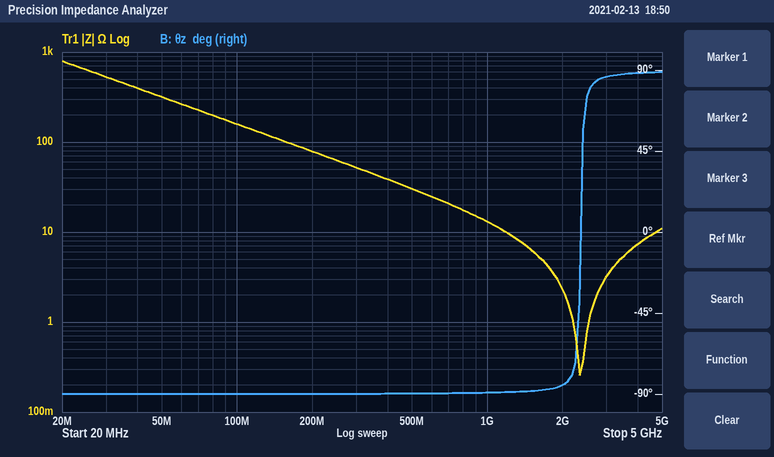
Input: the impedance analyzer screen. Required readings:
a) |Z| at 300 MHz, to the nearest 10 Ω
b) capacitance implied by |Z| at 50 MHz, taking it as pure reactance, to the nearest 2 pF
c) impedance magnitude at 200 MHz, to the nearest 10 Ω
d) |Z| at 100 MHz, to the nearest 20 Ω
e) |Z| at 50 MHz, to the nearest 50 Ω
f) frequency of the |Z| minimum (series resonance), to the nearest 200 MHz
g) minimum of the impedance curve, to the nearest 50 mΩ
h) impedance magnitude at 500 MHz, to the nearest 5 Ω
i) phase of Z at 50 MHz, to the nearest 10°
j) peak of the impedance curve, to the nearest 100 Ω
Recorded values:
50 Ω
10 pF
80 Ω
160 Ω
300 Ω
2.4 GHz
250 mΩ
30 Ω
-90°
800 Ω
